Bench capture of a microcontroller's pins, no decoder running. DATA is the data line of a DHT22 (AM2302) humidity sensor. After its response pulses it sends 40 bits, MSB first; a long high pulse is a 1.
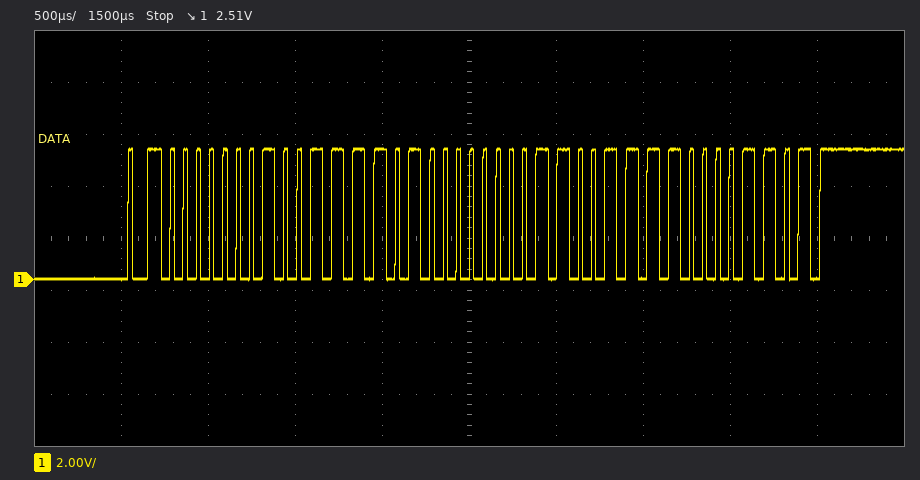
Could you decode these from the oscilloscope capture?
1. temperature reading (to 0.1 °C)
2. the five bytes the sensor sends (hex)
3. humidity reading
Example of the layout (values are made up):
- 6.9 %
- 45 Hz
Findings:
- 20.7 °C
- 01 3D 00 CF 0D
- 31.7 %
